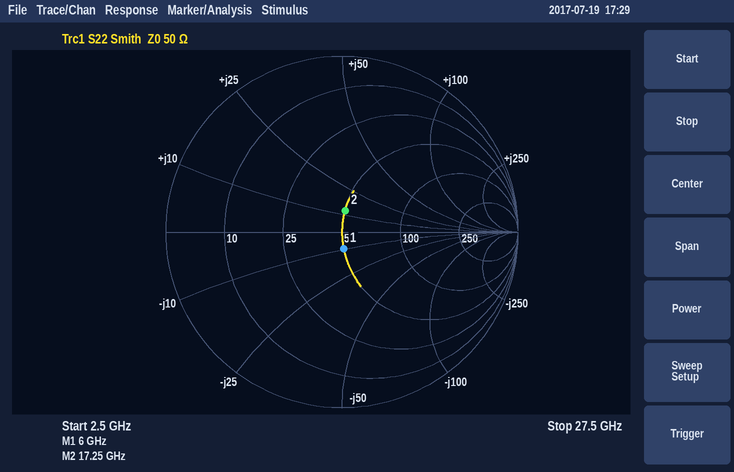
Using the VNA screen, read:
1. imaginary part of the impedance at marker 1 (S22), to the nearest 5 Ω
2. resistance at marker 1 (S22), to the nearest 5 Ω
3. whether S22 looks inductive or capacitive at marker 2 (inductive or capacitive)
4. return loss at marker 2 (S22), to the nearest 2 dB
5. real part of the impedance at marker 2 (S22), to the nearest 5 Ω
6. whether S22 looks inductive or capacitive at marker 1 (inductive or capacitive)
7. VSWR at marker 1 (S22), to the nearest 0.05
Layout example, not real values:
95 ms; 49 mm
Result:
-10 Ω; 50 Ω; inductive; 18 dB; 50 Ω; capacitive; 1.20
